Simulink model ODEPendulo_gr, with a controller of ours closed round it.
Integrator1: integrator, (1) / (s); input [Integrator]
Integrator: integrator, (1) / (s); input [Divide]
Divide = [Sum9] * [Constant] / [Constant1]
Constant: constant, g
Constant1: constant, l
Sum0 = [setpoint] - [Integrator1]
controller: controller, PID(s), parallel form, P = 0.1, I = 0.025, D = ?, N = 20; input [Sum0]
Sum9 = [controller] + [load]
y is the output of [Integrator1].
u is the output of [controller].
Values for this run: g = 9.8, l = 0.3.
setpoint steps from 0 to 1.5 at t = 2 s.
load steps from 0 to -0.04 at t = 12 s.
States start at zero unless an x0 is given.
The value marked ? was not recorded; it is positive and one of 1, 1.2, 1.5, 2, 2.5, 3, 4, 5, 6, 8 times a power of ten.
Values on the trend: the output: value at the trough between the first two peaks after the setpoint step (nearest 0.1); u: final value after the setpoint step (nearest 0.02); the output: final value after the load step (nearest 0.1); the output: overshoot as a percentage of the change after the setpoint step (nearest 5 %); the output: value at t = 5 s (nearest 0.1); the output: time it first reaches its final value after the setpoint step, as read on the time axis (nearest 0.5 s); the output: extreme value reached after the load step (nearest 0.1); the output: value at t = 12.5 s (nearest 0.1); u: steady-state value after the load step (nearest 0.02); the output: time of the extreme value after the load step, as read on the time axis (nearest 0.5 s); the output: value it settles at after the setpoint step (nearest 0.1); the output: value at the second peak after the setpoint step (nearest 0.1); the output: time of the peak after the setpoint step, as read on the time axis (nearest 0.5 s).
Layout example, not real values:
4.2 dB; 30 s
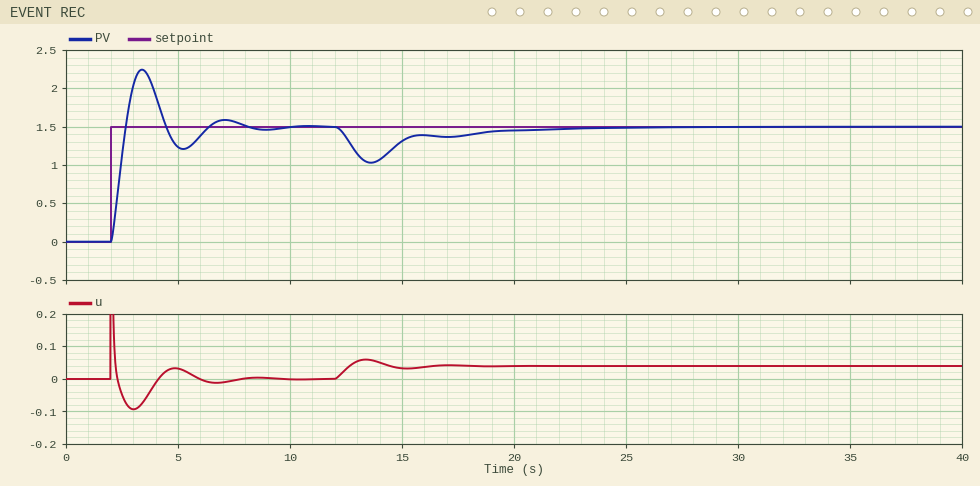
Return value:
1.2; 0.00; 1.5; 50 %; 1.2; 2.5 s; 1.0; 1.4; 0.04; 13.5 s; 1.5; 1.6; 3.5 s
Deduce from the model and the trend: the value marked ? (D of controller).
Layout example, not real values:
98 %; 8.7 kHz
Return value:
0.04
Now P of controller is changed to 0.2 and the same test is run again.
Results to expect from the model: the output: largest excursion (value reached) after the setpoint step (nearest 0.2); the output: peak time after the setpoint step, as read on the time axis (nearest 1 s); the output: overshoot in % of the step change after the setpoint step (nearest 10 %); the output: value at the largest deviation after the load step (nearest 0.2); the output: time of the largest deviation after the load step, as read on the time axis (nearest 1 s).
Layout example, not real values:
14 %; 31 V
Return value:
2.4; 3 s; 60 %; 1.2; 13 s
